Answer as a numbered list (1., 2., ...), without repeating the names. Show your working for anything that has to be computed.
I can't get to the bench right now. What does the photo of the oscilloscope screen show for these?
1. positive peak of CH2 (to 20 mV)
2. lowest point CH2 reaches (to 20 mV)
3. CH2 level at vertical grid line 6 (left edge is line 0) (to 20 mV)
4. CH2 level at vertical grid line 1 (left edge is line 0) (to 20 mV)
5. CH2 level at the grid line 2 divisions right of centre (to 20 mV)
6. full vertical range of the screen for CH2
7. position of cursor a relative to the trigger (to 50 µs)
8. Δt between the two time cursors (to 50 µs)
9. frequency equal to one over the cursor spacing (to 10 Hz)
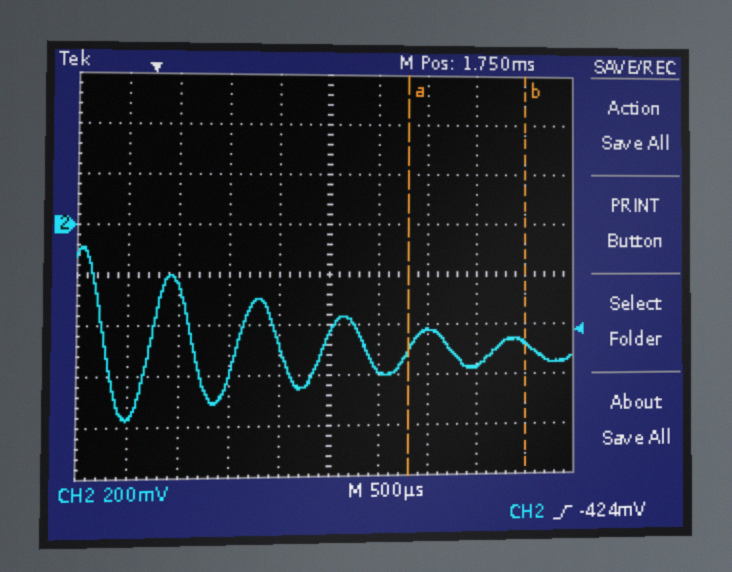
1. -80 mV
2. -780 mV
3. -580 mV
4. -760 mV
5. -420 mV
6. 1.6 V
7. +2.55 ms
8. 1.20 ms
9. 1 / 1.20 ms ≈ 830 Hz
